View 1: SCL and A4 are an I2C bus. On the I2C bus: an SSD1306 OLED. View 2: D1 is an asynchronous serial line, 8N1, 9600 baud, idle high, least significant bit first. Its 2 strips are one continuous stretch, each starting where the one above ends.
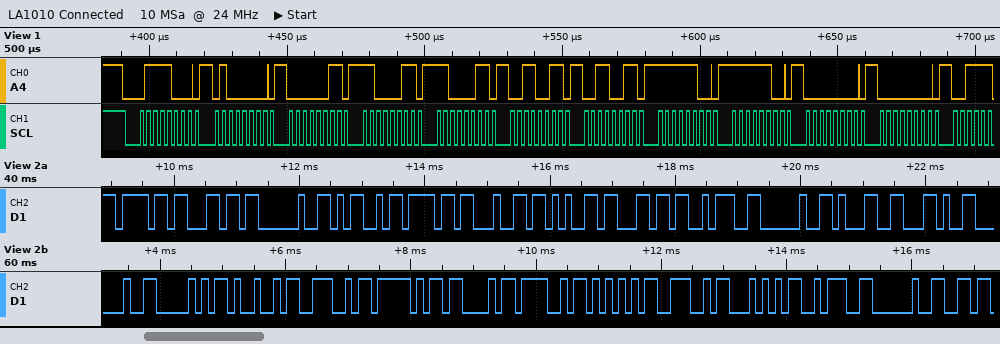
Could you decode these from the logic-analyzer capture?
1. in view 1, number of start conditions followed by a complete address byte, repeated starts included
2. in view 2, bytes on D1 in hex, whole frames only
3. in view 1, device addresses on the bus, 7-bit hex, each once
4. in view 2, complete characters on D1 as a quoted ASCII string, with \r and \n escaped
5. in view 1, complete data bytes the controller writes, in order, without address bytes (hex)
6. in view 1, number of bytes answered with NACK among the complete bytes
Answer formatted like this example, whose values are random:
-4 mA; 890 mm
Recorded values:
1; 6F 6C 20 4D 6F 64 65 6C 3A 20 31 2C 20 50 49 4E 5F 43 4F 55 4E 54 3A 20; 0x3C; "ol Model: 1, PIN_COUNT: "; 40 03 C3 C3 33 33 FC FC 00 00; 0
